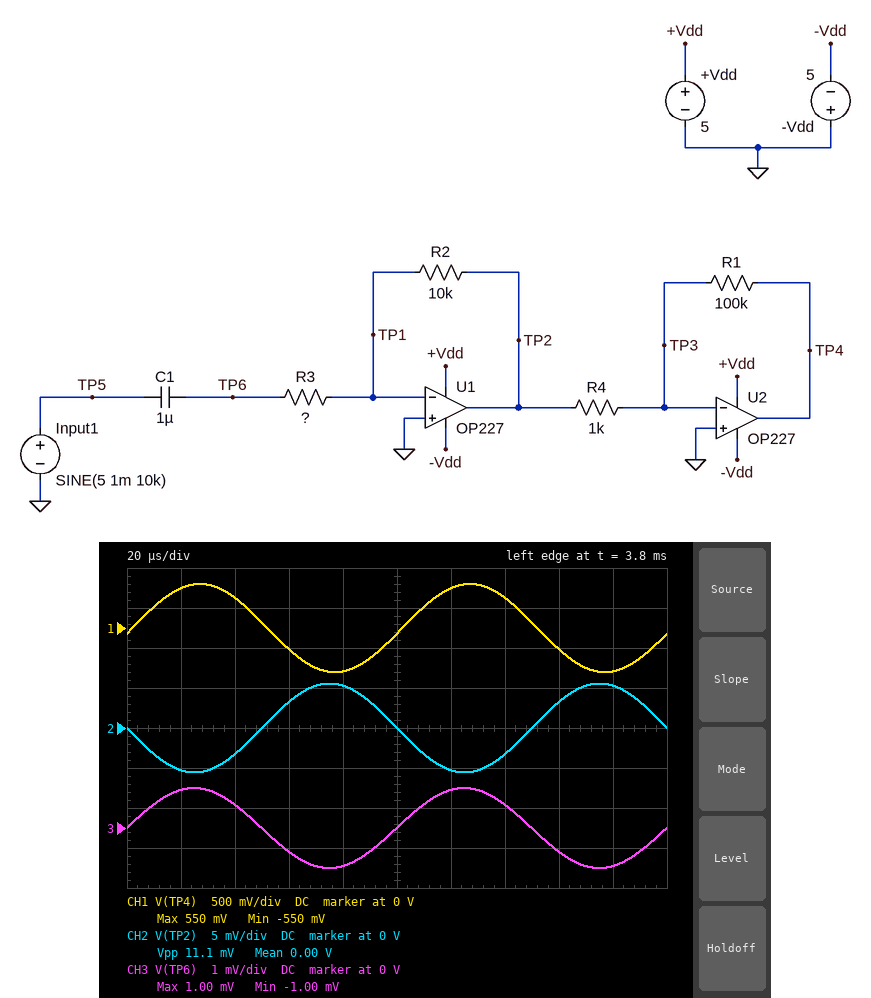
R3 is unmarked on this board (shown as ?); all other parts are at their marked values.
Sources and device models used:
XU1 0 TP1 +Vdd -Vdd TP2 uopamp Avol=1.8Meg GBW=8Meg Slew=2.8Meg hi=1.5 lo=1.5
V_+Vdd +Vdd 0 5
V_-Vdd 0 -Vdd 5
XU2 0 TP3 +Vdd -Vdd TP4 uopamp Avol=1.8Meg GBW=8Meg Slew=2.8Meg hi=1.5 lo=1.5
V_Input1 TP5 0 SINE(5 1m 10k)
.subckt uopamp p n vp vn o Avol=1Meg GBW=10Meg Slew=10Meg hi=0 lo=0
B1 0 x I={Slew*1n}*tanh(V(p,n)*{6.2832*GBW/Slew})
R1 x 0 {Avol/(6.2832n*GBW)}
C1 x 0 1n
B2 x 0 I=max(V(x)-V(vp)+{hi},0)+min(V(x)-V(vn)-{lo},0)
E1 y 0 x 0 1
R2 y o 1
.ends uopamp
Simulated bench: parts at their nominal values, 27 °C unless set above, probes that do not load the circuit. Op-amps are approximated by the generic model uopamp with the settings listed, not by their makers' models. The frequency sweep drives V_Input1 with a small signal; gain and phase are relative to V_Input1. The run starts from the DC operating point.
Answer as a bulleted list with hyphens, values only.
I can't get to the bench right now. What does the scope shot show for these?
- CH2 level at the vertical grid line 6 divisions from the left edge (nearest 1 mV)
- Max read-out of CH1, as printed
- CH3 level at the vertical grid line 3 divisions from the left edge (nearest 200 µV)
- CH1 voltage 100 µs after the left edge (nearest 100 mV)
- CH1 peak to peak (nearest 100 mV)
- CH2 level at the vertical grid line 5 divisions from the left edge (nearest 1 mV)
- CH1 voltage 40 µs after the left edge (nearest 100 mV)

- -5 mV
- 550 mV
- -600 µV
- -100 mV
- 1.1 V
- 0 V
- 400 mV
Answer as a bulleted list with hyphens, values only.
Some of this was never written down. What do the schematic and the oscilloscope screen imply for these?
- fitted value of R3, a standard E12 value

- 1.8 kΩ
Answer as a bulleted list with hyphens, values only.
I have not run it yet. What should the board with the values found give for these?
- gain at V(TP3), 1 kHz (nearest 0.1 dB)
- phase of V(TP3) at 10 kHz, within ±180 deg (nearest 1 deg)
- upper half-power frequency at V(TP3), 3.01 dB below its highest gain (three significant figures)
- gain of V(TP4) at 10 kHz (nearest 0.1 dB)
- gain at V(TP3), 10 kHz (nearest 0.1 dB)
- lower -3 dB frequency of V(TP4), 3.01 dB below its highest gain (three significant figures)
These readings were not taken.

- -23.2 dB
- -97 deg
- 1.37 MHz
- 54.8 dB
- -3.2 dB
- 88.2 Hz
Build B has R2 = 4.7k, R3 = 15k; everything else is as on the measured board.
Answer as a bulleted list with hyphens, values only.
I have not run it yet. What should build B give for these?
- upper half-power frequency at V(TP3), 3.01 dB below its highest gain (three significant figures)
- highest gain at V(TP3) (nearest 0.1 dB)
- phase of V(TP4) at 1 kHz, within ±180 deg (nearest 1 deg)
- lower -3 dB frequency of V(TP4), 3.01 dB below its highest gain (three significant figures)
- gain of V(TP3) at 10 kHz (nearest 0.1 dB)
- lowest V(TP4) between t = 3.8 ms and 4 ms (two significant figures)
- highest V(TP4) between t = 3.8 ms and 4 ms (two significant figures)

- 6.25 MHz
- -10.3 dB
- 0 deg
- 10.6 Hz
- -28.2 dB
- -31 mV
- 31 mV
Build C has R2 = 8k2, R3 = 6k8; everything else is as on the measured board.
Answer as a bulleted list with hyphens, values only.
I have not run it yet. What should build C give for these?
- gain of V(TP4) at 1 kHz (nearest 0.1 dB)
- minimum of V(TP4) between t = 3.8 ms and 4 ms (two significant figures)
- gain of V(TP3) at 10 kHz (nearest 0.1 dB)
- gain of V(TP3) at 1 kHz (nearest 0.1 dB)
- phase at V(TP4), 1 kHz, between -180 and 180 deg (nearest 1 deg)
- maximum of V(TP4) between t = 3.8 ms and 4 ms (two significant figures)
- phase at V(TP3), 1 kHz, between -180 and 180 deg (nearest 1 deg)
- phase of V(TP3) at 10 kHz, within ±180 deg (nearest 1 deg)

- 41.6 dB
- -120 mV
- -16.5 dB
- -36.4 dB
- 1 deg
- 120 mV
- -90 deg
- -97 deg
